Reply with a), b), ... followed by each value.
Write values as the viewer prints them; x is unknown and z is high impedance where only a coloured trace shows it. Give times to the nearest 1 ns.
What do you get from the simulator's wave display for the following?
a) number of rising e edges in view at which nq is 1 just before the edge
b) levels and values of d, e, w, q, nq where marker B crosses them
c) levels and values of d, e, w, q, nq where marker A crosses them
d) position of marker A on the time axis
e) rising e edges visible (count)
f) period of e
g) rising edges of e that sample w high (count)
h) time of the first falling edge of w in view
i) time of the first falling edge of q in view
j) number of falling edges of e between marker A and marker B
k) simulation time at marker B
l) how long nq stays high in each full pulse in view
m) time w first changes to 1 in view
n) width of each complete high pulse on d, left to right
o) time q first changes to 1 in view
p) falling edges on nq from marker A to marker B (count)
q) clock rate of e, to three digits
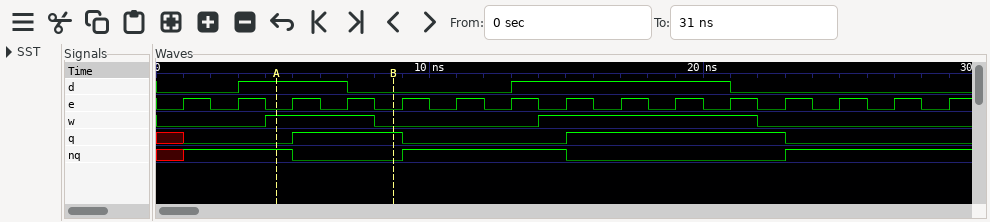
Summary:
a) 8
b) d=0, e=0, w=0, q=1, nq=0
c) d=1, e=0, w=1, q=0, nq=1
d) 4 ns
e) 15
f) 2 ns
g) 6
h) 8 ns
i) 9 ns
j) 2
k) 9 ns
l) 6 ns
m) 4 ns
n) 4 ns, 8 ns
o) 5 ns
p) 1
q) 500 MHz
